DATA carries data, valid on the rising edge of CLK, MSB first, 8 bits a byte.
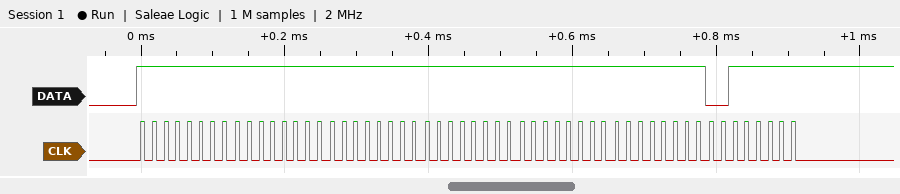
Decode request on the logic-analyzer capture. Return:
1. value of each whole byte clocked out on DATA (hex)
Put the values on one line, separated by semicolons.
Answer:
FF FF FF FF FF FF 3F
